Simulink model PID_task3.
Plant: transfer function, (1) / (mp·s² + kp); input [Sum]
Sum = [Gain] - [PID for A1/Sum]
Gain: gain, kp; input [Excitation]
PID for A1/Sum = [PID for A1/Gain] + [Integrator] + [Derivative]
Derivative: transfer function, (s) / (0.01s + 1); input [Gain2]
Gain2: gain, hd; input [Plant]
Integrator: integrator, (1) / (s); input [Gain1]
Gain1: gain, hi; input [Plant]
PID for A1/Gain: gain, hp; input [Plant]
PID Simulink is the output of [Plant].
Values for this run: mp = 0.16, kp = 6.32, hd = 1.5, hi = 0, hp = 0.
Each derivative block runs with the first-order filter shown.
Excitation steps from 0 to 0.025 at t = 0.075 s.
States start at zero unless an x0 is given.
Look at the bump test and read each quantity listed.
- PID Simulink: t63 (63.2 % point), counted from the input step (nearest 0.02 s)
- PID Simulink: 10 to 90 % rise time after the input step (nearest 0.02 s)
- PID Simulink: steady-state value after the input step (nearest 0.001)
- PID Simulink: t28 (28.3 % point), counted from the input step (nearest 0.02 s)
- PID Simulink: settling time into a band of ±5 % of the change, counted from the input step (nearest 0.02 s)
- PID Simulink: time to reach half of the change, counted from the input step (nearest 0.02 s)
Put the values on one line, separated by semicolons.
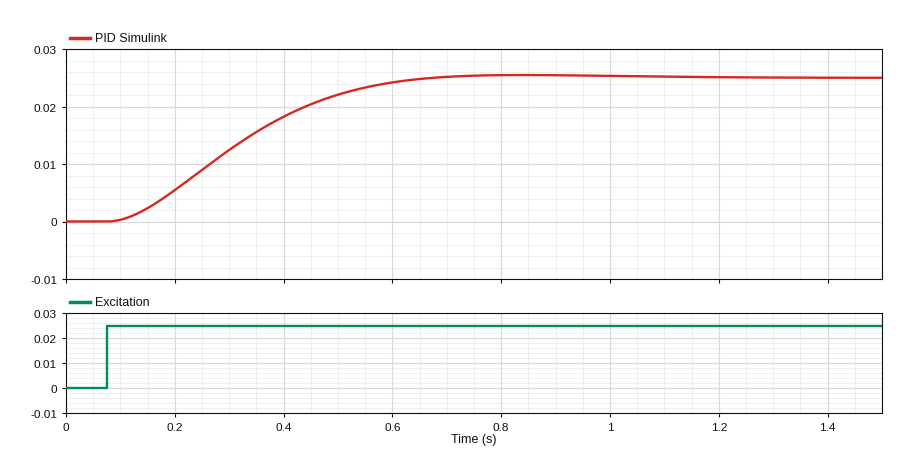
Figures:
0.28 s; 0.36 s; 0.025; 0.14 s; 0.50 s; 0.22 s
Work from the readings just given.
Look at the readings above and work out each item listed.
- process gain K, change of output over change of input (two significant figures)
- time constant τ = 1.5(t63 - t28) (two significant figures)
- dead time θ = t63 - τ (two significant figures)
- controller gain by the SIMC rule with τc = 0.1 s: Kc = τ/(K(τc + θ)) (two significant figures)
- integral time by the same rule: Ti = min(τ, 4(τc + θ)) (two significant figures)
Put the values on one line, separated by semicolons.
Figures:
1.0; 0.21 s; 0.070 s; 1.2; 0.21 s
